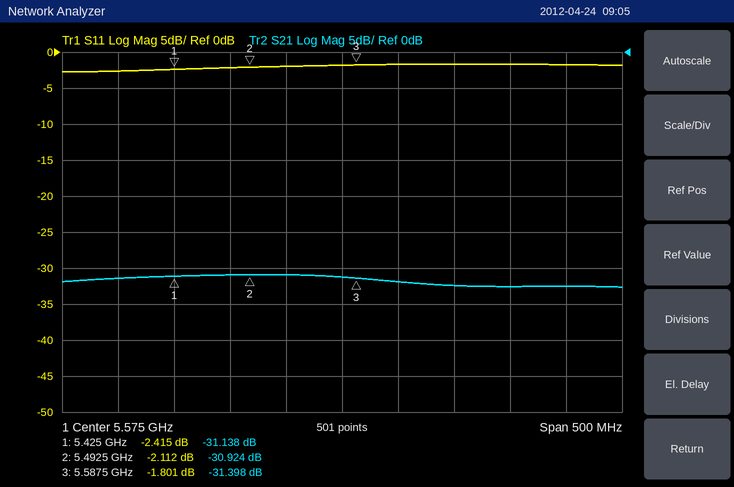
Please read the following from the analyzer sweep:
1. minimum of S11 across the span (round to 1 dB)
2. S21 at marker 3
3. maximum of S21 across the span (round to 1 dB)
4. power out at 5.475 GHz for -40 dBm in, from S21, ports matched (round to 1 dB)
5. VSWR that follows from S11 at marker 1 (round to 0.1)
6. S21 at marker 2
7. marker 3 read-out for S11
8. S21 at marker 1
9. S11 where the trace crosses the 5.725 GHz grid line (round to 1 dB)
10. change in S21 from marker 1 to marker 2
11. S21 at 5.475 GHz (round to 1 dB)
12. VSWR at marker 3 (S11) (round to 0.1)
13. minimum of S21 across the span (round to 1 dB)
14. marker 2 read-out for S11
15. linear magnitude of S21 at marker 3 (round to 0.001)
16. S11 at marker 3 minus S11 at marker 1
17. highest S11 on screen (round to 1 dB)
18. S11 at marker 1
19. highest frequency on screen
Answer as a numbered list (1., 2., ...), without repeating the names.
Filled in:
1. -3 dB
2. -31.398 dB
3. -31 dB
4. -71 dBm
5. 7.2
6. -30.924 dB
7. -1.801 dB
8. -31.138 dB
9. -2 dB
10. 0.214 dB
11. -31 dB
12. 9.7
13. -33 dB
14. -2.112 dB
15. 0.027
16. 0.614 dB
17. -2 dB
18. -2.415 dB
19. 5.825 GHz
